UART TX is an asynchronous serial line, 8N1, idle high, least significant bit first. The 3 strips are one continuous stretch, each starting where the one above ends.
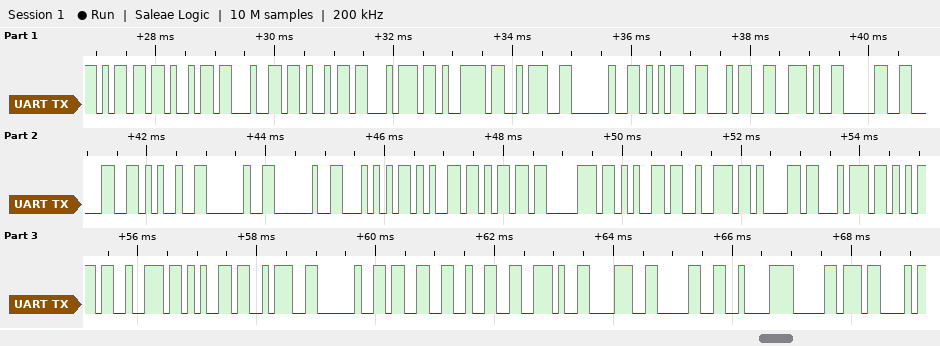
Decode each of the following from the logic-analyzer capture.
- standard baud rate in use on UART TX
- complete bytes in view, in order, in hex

9600 baud
0x6D 0x69 0x64 0x69 0x74 0x79 0x3A 0x20 0x35 0x34 0x2E 0x30 0x30 0x25 0x20 0x20 0x54 0x65 0x6D 0x70 0x65 0x72 0x61 0x74 0x75 0x72 0x65 0x3A 0x20 0x33 0x32 0x2E 0x38 0x30 0xC2 0xB0 0x43
